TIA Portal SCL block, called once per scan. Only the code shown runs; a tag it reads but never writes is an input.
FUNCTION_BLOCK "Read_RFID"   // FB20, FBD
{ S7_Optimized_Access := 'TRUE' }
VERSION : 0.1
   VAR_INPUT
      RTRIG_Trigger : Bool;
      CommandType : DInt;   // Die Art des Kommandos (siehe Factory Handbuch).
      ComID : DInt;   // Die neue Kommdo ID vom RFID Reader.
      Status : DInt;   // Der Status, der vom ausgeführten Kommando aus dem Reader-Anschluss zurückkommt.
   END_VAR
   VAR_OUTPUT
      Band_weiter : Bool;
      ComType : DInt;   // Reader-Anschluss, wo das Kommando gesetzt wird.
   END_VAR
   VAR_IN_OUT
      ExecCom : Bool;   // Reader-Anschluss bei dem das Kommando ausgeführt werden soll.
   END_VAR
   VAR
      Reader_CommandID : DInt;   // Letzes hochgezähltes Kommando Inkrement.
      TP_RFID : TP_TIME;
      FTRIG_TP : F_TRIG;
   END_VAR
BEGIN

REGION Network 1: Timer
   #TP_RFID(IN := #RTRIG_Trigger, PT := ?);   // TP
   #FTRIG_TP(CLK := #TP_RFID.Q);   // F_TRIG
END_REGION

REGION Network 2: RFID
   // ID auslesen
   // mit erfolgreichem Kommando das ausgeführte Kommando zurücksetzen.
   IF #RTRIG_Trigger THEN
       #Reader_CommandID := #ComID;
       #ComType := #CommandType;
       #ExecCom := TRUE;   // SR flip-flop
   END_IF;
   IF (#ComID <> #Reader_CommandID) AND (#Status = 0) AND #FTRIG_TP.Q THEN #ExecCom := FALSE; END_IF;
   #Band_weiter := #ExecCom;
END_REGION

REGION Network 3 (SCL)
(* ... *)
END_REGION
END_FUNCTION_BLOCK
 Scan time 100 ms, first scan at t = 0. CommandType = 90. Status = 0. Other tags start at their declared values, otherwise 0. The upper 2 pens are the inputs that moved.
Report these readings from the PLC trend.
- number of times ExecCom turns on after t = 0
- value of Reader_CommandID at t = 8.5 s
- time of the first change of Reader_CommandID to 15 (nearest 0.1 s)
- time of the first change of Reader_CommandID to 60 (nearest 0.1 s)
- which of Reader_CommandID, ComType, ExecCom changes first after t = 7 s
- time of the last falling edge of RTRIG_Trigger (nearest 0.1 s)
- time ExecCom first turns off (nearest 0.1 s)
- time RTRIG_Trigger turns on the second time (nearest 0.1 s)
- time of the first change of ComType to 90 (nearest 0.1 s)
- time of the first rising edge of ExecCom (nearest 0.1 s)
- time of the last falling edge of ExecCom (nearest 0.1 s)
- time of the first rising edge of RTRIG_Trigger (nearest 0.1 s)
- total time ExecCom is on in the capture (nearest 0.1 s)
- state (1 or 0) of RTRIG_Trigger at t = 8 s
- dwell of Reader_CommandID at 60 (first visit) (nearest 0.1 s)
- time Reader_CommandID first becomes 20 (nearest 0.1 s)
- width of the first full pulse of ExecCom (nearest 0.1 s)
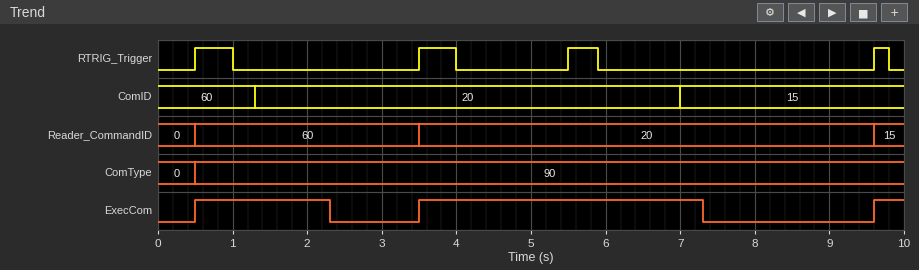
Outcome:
3
20
9.6 s
0.5 s
ExecCom
9.8 s
2.3 s
3.5 s
0.5 s
0.5 s
7.3 s
0.5 s
6.0 s
0
3.0 s
3.5 s
1.8 s
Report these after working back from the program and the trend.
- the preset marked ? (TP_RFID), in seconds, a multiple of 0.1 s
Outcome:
1.8 s
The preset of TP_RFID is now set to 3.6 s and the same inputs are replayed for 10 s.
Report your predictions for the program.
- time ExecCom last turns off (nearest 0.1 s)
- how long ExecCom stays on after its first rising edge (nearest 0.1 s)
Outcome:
9.1 s
8.6 s
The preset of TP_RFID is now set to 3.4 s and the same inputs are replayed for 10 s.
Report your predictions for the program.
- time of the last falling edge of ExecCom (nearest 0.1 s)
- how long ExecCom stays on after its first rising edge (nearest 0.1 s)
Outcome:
8.9 s
8.4 s
